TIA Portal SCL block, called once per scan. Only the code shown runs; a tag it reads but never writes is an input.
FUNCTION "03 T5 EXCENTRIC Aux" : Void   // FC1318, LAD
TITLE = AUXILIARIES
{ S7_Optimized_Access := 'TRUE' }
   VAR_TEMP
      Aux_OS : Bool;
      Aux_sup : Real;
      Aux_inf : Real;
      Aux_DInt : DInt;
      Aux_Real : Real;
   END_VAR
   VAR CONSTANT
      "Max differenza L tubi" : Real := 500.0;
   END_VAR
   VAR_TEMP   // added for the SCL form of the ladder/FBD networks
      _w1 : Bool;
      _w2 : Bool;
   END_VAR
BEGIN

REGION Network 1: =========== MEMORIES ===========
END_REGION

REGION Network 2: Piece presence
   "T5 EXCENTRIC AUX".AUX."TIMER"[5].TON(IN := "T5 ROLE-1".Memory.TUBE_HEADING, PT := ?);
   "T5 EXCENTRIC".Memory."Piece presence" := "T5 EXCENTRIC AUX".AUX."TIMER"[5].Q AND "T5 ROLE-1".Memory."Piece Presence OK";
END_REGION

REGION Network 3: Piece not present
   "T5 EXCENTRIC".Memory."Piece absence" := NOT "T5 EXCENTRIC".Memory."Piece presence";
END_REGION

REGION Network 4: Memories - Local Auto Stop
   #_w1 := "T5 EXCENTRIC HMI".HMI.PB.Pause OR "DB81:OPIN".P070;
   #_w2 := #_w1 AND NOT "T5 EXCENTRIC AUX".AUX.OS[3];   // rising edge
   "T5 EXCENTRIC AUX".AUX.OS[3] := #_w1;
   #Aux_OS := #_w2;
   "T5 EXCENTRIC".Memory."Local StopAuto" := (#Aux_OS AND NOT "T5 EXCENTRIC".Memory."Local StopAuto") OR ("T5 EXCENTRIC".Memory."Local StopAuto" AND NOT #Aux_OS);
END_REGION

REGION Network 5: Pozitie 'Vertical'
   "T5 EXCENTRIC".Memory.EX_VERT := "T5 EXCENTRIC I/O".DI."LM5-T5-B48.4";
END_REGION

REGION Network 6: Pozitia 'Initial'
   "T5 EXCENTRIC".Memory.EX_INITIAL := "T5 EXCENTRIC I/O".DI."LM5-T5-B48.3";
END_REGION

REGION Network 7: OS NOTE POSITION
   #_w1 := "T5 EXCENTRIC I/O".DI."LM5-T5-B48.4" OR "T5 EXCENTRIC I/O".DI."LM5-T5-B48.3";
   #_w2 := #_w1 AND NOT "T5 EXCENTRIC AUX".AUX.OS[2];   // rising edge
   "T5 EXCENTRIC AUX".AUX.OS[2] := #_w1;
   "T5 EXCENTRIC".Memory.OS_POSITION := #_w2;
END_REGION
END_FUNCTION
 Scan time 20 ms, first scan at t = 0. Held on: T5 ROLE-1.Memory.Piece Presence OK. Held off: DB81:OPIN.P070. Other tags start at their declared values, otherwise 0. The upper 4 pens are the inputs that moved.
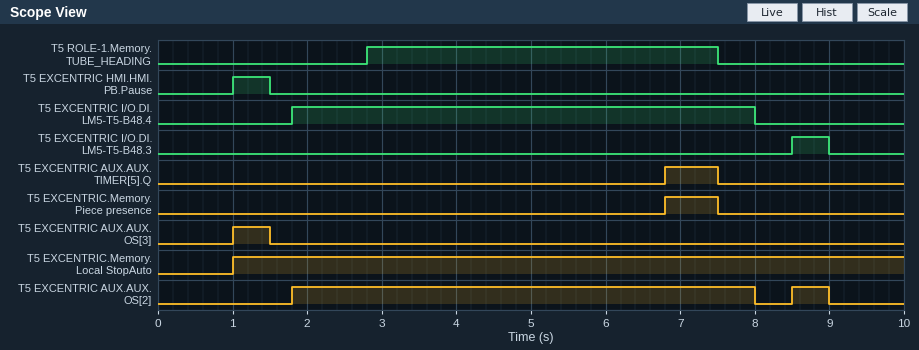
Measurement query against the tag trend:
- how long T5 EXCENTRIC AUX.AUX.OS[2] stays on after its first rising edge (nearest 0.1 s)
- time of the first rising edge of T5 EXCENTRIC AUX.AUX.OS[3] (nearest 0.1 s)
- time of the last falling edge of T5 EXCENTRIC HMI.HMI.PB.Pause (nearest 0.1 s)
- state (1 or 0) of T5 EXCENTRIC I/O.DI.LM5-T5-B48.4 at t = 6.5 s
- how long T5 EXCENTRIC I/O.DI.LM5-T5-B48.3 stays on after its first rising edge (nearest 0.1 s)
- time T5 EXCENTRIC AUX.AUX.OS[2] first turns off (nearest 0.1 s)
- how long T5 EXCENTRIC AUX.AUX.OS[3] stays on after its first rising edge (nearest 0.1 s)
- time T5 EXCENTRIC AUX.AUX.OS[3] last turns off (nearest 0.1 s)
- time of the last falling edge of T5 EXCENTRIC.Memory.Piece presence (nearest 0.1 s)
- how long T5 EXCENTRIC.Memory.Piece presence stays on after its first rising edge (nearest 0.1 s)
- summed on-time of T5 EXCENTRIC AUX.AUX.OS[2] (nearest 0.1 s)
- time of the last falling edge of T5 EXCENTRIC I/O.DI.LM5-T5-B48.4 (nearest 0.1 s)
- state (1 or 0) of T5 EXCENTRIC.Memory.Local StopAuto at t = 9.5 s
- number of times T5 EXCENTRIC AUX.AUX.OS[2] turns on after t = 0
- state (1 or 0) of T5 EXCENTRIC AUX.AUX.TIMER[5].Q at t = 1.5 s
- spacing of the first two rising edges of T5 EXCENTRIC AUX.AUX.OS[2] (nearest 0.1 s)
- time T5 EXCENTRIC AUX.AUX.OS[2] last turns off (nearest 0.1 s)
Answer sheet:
6.2 s
1.0 s
1.5 s
1
0.5 s
8.0 s
0.5 s
1.5 s
7.5 s
0.7 s
6.7 s
8.0 s
1
2
0
6.7 s
9.0 s
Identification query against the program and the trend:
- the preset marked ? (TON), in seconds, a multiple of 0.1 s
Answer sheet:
4.0 s
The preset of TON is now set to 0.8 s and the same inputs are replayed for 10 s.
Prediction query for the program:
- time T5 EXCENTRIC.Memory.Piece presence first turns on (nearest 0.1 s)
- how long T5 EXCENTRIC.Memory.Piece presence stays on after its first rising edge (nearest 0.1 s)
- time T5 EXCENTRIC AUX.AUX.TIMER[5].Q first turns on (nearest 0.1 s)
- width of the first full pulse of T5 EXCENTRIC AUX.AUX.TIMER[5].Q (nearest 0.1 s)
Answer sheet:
3.6 s
3.9 s
3.6 s
3.9 s
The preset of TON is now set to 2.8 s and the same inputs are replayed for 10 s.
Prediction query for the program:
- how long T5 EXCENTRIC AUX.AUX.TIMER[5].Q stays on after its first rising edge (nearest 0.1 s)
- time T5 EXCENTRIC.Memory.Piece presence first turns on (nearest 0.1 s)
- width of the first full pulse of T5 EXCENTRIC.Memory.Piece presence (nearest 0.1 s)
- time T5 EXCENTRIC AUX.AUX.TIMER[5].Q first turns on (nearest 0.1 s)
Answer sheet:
1.9 s
5.6 s
1.9 s
5.6 s
